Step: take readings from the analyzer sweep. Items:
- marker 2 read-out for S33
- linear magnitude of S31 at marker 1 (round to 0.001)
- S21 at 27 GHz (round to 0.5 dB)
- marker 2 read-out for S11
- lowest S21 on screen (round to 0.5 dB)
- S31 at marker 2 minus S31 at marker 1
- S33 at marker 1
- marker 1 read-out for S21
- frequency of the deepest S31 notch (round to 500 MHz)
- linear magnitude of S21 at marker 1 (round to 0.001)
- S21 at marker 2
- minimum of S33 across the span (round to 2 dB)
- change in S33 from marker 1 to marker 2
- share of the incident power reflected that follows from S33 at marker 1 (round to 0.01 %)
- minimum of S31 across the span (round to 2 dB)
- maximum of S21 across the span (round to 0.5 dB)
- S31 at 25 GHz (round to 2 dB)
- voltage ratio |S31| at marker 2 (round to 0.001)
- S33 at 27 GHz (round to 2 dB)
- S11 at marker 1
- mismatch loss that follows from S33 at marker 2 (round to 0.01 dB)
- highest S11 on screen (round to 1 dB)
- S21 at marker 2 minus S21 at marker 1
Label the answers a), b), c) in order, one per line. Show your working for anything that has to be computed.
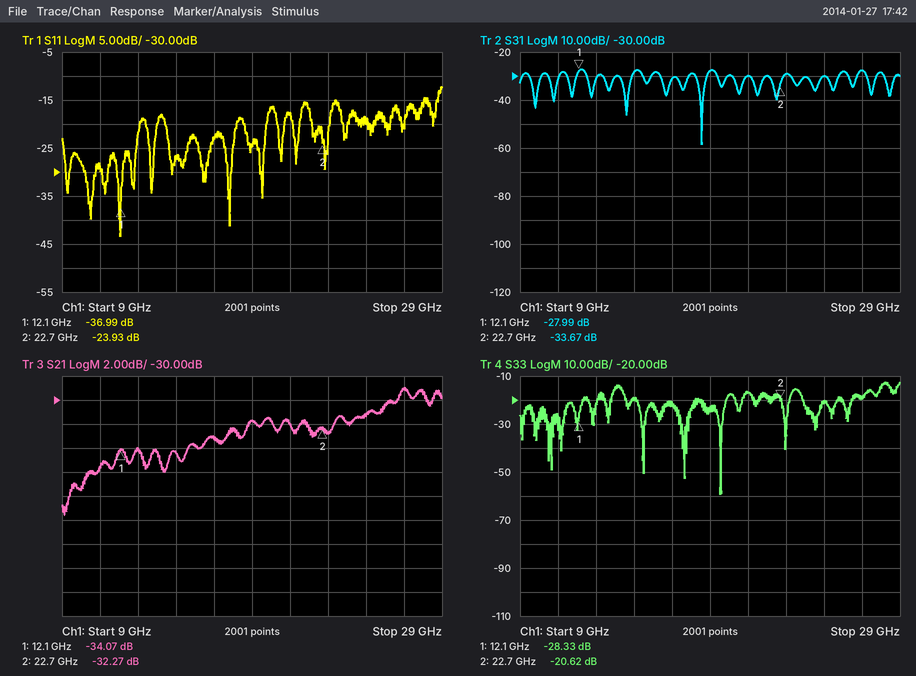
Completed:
a) -20.62 dB
b) 10^(-27.99/20) ≈ 0.040
c) -29.0 dB
d) -23.93 dB
e) -39.5 dB
f) -33.67 − (-27.99) = -5.68 dB
g) -28.33 dB
h) -34.07 dB
i) 18.5 GHz
j) 10^(-34.07/20) ≈ 0.020
k) -32.27 dB
l) -60 dB
m) -20.62 − (-28.33) = 7.71 dB
n) 10^(-28.33/10) ≈ 0.15 %
o) -58 dB
p) -29.0 dB
q) -30 dB
r) 10^(-33.67/20) ≈ 0.021
s) -18 dB
t) -36.99 dB
u) −10 log10(1 − 10^(-20.62/10)) ≈ 0.04 dB
v) -12 dB
w) -32.27 − (-34.07) = 1.80 dB
